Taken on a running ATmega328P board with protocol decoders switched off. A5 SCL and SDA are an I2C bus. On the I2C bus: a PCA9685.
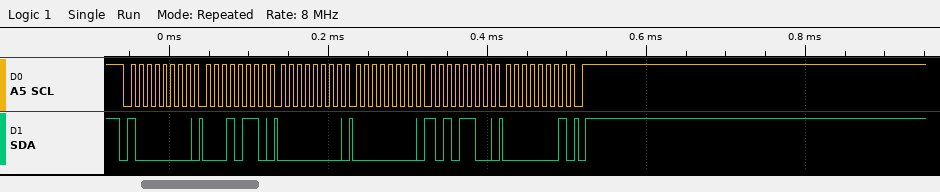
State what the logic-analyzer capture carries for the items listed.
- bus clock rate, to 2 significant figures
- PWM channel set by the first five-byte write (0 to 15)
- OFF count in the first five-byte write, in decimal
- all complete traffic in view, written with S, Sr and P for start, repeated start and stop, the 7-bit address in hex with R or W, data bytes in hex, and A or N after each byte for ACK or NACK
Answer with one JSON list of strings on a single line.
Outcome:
["100 kHz", "4", "428", "S 40W A 16 A 00 A 00 A AC A 01 A P"]
